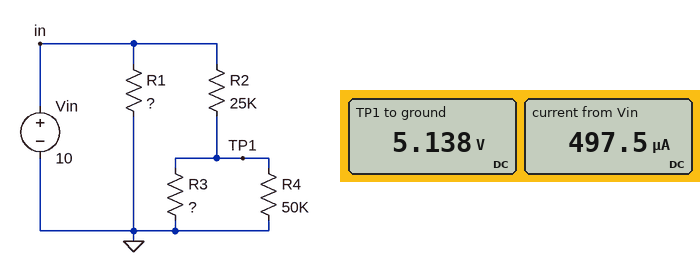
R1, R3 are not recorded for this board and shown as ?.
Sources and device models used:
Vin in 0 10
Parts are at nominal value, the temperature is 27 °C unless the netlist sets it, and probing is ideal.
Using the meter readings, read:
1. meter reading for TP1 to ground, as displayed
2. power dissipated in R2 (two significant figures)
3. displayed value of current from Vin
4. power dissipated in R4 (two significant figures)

5.138 V
950 µW
497.5 µA
530 µW
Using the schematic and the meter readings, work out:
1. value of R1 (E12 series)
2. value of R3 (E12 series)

33 kΩ
56 kΩ
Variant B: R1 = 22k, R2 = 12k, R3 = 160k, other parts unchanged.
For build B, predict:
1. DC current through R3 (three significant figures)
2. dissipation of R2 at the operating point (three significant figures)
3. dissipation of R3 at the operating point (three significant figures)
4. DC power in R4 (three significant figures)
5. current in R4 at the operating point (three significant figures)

47.5 µA
478 µW
361 µW
1.16 mW
152 µA
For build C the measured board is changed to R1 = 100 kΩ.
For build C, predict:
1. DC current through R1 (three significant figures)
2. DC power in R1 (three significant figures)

100 µA
1.00 mW
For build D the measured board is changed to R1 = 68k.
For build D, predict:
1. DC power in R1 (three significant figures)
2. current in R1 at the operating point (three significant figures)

1.47 mW
147 µA
